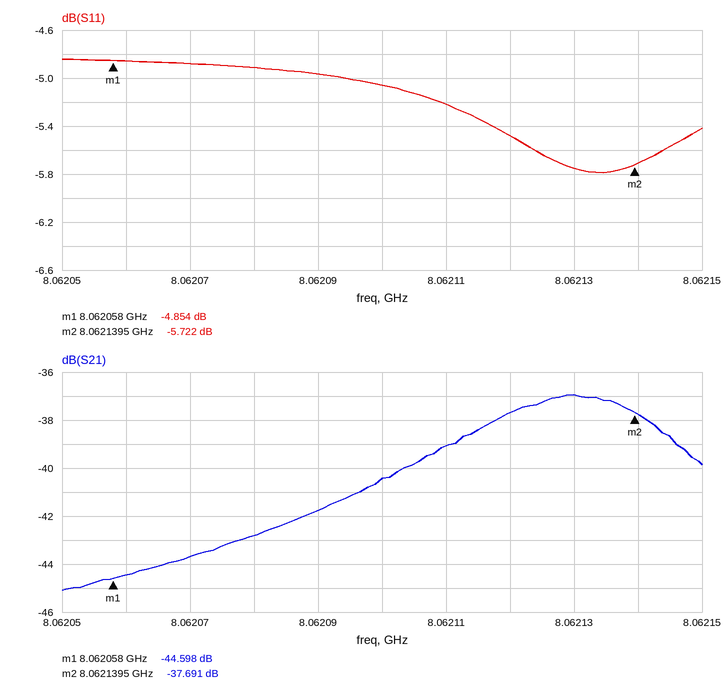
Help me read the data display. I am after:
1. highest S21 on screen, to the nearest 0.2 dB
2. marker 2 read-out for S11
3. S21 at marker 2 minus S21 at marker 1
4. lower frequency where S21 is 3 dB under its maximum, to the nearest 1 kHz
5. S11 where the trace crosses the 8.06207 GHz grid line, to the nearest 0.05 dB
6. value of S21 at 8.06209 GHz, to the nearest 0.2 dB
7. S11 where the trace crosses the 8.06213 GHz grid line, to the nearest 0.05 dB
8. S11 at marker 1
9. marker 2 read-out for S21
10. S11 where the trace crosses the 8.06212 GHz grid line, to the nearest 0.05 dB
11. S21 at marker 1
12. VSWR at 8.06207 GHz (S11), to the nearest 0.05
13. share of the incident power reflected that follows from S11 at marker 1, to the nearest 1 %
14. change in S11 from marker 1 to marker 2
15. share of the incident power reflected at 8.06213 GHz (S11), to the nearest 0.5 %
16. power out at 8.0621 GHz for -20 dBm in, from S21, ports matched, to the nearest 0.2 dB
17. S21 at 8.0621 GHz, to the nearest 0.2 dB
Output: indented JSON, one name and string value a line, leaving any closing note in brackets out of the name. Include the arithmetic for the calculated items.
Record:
{
  "highest S21 on screen, to the nearest 0.2 dB": "-37.0 dB",
  "marker 2 read-out for S11": "-5.722 dB",
  "S21 at marker 2 minus S21 at marker 1": "-37.691 − (-44.598) = 6.907 dB",
  "lower frequency where S21 is 3 dB under its maximum, to the nearest 1 kHz": "8.062104 GHz",
  "S11 where the trace crosses the 8.06207 GHz grid line, to the nearest 0.05 dB": "-4.90 dB",
  "value of S21 at 8.06209 GHz, to the nearest 0.2 dB": "-41.8 dB",
  "S11 where the trace crosses the 8.06213 GHz grid line, to the nearest 0.05 dB": "-5.75 dB",
  "S11 at marker 1": "-4.854 dB",
  "marker 2 read-out for S21": "-37.691 dB",
  "S11 where the trace crosses the 8.06212 GHz grid line, to the nearest 0.05 dB": "-5.50 dB",
  "S21 at marker 1": "-44.598 dB",
  "VSWR at 8.06207 GHz (S11), to the nearest 0.05": "|Γ| = 10^(-4.9/20) = 0.5689; VSWR = (1 + 0.5689)/(1 − 0.5689) ≈ 3.64, so 3.65 to the nearest 0.05",
  "share of the incident power reflected that follows from S11 at marker 1, to the nearest 1 %": "10^(-4.854/10) ≈ 33 %",
  "change in S11 from marker 1 to marker 2": "-5.722 − (-4.854) = -0.868 dB",
  "share of the incident power reflected at 8.06213 GHz (S11), to the nearest 0.5 %": "10^(-5.75/10) ≈ 26.6 %, so 26.5 % to the nearest 0.5 %",
  "power out at 8.0621 GHz for -20 dBm in, from S21, ports matched, to the nearest 0.2 dB": "-20 dBm + (-40.4 dB) = -60.4 dBm",
  "S21 at 8.0621 GHz, to the nearest 0.2 dB": "-40.4 dB"
}
